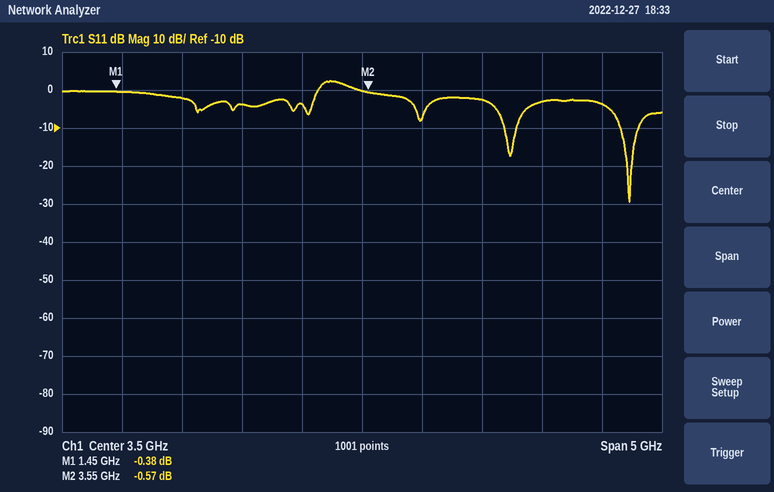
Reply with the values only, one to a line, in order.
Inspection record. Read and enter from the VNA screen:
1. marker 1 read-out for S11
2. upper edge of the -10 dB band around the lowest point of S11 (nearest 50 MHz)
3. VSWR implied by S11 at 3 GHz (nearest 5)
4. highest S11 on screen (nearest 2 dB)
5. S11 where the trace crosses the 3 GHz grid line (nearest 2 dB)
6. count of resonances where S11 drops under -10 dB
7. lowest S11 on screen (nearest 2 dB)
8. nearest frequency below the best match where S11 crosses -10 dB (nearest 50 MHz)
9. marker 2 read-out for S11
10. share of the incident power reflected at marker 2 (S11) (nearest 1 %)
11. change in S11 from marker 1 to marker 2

-0.38 dB
5.80 GHz
5
2 dB
-4 dB
2
-30 dB
5.65 GHz
-0.57 dB
88 %
-0.19 dB
